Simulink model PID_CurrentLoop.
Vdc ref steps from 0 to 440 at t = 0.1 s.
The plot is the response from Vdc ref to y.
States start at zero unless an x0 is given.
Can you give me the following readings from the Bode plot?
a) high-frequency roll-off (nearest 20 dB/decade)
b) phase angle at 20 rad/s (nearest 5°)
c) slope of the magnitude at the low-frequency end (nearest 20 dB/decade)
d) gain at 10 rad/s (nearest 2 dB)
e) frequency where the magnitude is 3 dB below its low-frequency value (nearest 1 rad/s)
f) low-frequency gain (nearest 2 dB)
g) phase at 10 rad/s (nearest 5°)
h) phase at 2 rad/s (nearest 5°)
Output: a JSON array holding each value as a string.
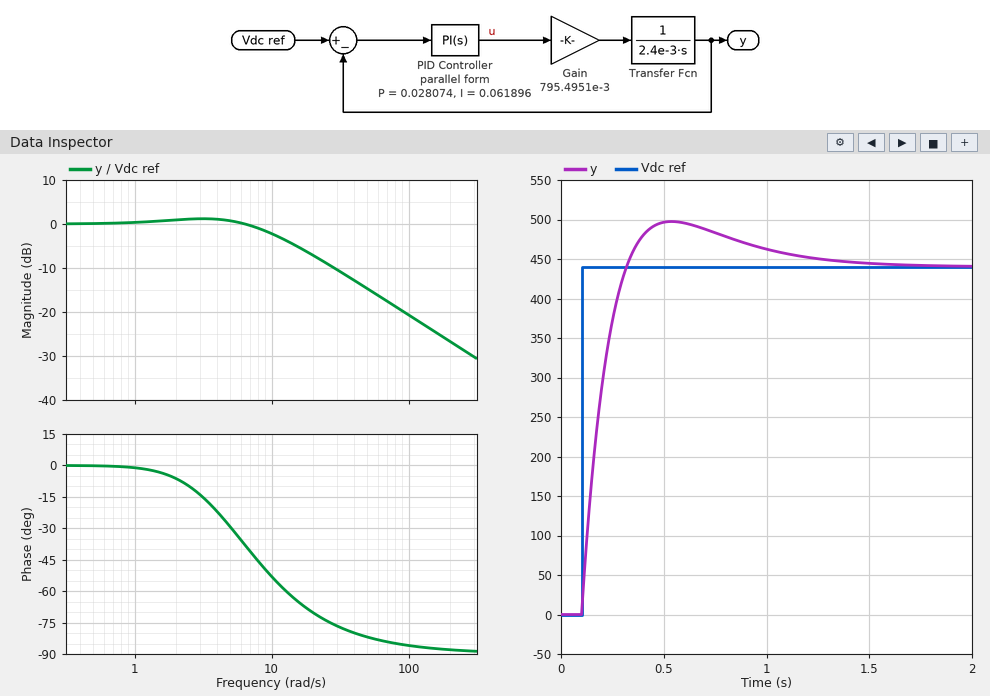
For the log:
["-20 dB/decade", "-70°", "0 dB/decade", "-2 dB", "11 rad/s", "0 dB", "-55°", "-5°"]
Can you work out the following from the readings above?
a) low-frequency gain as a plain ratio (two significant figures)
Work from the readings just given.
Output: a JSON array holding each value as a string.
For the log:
["1.0"]
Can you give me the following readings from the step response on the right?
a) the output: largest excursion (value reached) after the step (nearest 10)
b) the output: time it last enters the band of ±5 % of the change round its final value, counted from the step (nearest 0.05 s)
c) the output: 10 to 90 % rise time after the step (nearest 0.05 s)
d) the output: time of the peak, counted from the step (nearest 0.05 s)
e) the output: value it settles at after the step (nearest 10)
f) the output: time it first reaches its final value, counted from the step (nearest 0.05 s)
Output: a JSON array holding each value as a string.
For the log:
["500", "0.90 s", "0.15 s", "0.45 s", "440", "0.20 s"]
